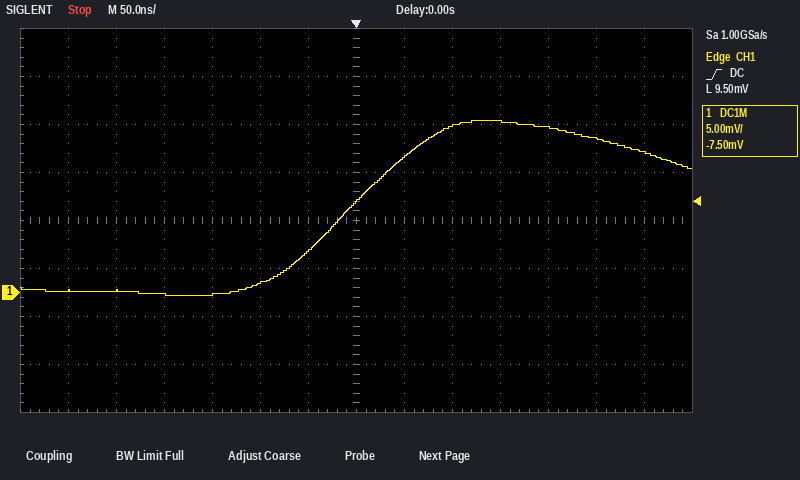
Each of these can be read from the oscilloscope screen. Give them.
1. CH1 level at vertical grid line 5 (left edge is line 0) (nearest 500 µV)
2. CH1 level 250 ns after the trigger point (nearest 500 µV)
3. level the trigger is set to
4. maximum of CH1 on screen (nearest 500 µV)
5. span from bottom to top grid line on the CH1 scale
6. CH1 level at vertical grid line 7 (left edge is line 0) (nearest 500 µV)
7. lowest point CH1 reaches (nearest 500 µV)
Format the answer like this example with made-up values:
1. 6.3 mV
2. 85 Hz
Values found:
1. 1.0 mV
2. 16.0 mV
3. 9.50 mV
4. 18.0 mV
5. 40 mV
6. 9.5 mV
7. -500 µV
